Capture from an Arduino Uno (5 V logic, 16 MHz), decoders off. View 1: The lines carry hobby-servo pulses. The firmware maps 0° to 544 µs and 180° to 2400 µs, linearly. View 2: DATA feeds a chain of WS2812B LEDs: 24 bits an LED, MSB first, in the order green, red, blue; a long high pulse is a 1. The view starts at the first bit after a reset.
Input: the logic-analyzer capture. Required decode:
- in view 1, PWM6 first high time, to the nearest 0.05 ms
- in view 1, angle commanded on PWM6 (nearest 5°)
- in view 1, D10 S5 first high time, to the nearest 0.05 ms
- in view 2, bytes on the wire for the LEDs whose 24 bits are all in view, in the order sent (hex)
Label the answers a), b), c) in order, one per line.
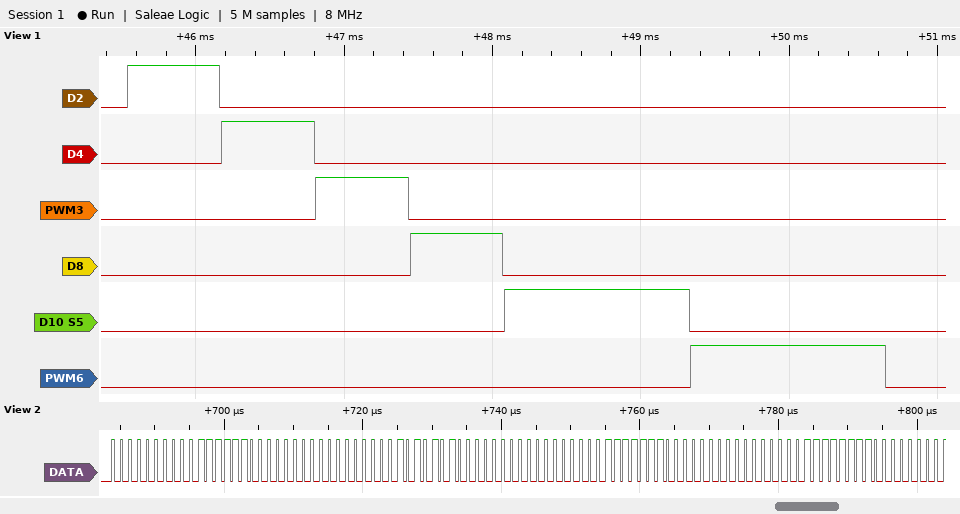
a) 1.30 ms
b) 75°
c) 1.25 ms
d) 00 3F 00 00 55 00 00 7F 00 00 FF 00
